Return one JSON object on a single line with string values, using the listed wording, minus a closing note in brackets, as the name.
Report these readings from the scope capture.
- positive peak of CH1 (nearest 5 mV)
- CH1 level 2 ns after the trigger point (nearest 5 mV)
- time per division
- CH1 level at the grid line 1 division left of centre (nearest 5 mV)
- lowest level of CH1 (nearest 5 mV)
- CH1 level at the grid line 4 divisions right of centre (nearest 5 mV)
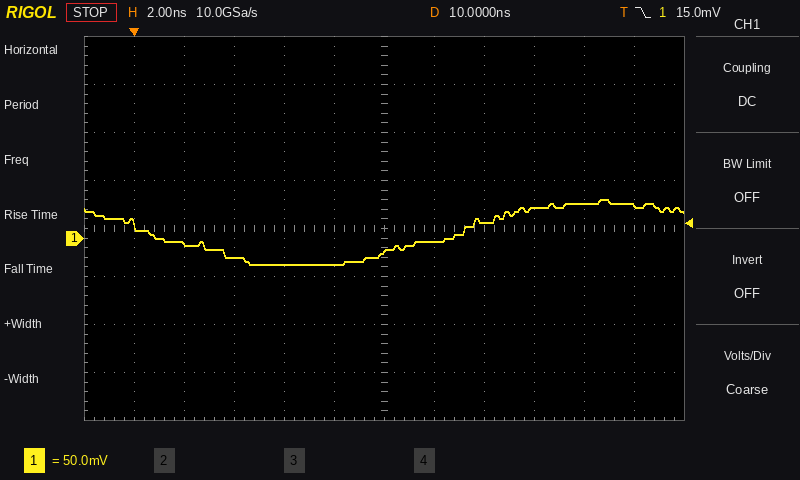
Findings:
{"positive peak of CH1": "40 mV", "CH1 level 2 ns after the trigger point": "-5 mV", "time per division": "2 ns", "CH1 level at the grid line 1 division left of centre": "-30 mV", "lowest level of CH1": "-30 mV", "CH1 level at the grid line 4 divisions right of centre": "35 mV"}
